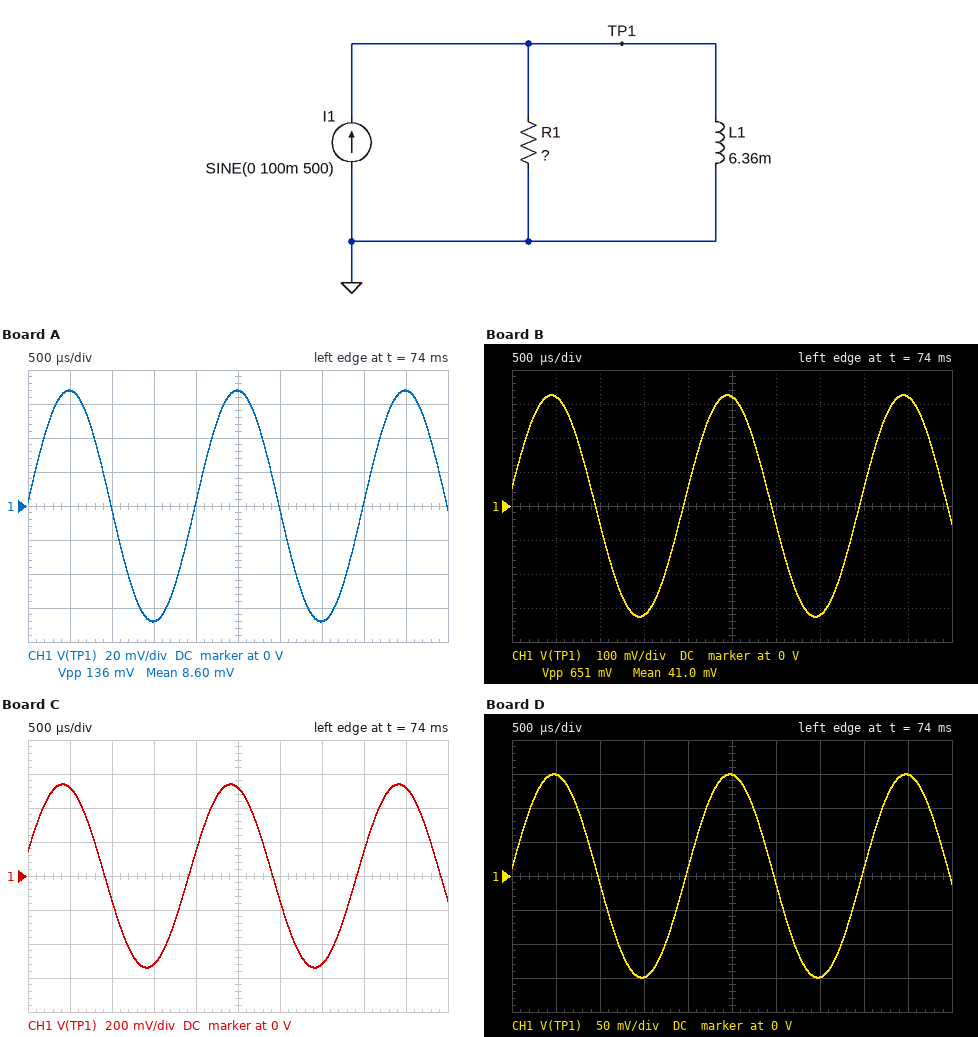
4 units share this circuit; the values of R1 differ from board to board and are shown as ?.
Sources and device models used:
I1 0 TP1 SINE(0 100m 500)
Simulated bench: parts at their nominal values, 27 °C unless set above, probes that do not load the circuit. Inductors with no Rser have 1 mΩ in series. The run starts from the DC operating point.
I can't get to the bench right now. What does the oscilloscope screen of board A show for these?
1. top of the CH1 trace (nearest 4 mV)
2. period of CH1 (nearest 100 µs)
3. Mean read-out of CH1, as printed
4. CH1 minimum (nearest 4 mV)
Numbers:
68 mV
2.0 ms
8.60 mV
-68 mV
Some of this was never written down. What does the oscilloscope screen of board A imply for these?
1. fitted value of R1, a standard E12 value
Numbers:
0.68 Ω
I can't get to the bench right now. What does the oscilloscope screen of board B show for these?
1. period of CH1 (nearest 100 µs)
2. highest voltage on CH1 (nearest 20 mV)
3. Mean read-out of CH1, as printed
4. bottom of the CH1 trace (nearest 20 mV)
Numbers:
2.0 ms
320 mV
41.0 mV
-320 mV
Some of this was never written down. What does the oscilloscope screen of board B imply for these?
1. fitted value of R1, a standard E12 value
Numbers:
3.3 Ω
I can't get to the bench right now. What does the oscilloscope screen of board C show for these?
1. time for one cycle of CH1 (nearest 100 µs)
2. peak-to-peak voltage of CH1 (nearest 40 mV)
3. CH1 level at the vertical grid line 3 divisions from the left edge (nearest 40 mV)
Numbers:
2.0 ms
1.08 V
-520 mV
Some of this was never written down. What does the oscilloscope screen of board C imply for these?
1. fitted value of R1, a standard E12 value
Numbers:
5.6 Ω
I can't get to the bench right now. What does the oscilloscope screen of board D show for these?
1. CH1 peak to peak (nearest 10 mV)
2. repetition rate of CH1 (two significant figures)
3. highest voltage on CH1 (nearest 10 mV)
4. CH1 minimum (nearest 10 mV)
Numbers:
300 mV
500 Hz
150 mV
-150 mV
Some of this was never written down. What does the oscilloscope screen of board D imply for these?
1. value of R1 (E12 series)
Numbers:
1.5 Ω
